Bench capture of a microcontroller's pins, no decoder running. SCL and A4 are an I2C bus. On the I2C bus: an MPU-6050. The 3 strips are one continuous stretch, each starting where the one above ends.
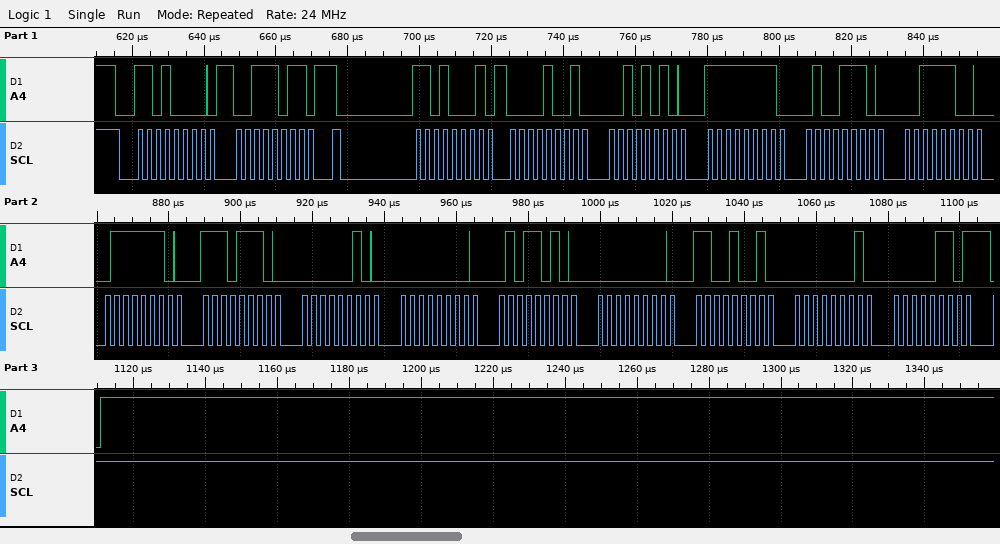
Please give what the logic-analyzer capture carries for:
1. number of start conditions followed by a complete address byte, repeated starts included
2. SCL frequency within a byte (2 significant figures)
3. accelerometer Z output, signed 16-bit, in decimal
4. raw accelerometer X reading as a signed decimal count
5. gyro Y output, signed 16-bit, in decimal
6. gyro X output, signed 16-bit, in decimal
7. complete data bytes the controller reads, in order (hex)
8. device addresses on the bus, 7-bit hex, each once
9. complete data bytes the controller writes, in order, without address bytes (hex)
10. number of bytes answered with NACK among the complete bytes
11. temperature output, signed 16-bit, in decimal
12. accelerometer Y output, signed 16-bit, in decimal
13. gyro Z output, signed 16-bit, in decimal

2
400 kHz
15486
2346
201
90
09 2A FF 4E 3C 7E EE 02 00 5A 00 C9 01 06
0x68
3B
1
-4606
-178
262
